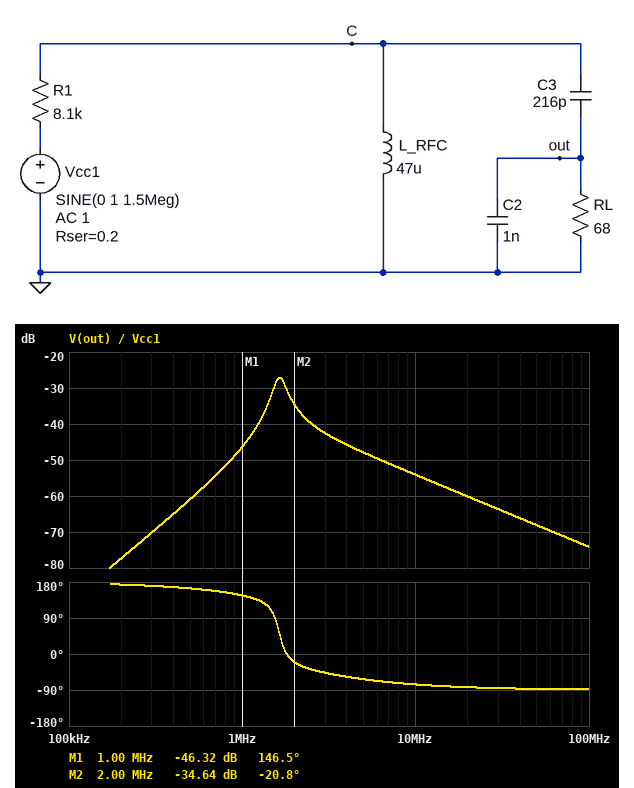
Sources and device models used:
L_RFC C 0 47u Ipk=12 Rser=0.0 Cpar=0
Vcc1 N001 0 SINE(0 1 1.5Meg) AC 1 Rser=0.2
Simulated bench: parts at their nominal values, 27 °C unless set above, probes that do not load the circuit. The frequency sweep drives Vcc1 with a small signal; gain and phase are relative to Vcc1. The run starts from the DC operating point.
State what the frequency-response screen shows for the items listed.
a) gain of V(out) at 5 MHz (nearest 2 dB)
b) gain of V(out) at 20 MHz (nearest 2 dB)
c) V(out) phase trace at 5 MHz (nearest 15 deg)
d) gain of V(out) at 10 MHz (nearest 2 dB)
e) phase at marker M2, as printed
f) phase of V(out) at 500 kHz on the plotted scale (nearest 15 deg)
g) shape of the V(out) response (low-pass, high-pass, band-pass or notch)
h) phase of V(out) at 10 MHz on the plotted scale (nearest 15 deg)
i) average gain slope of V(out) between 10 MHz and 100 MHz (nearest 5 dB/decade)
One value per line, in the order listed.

-48 dB
-60 dB
-60 deg
-54 dB
-20.8 deg
165 deg
band-pass
-75 deg
-20 dB/decade
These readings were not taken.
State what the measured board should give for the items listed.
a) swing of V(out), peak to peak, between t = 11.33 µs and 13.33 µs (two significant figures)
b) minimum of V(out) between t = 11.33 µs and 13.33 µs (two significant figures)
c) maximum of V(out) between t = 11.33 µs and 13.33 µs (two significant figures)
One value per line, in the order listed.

58 mV
-29 mV
29 mV
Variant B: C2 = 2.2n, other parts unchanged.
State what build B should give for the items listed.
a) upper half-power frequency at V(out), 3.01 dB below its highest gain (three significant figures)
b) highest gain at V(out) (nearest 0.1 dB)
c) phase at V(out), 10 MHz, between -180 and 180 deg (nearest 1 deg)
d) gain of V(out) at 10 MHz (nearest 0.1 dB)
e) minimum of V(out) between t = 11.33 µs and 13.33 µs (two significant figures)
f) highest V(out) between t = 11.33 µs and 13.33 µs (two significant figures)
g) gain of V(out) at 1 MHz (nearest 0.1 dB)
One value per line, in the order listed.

1.72 MHz
-26.9 dB
-83 deg
-60.8 dB
-23 mV
23 mV
-48.5 dB
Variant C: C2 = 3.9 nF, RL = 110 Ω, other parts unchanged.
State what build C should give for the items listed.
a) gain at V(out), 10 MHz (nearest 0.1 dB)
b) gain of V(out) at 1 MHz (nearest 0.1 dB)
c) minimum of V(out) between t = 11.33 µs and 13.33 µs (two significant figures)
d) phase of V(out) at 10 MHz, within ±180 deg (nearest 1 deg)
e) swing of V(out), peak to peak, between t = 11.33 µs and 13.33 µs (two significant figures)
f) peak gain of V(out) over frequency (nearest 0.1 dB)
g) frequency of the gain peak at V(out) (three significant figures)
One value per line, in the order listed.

-65.7 dB
-50.7 dB
-18 mV
-87 deg
36 mV
-27.3 dB
1.62 MHz
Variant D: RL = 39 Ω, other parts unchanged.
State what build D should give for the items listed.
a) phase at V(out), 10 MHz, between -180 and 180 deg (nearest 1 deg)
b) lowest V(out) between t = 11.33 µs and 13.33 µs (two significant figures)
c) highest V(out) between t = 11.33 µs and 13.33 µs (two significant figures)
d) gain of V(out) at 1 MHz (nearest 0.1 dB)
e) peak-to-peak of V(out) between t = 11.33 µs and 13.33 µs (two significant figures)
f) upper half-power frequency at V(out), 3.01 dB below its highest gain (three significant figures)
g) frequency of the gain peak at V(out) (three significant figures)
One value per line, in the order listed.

-67 deg
-23 mV
23 mV
-50.3 dB
47 mV
1.72 MHz
1.61 MHz
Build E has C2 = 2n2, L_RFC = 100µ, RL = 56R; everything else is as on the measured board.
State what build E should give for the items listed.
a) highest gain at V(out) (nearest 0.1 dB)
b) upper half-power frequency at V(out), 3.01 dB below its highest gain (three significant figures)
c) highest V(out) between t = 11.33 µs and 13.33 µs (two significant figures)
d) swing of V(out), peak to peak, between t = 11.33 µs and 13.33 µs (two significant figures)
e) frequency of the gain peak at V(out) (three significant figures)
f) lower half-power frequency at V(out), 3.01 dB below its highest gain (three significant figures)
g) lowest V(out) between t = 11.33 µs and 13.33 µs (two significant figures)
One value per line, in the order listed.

-28.0 dB
1.19 MHz
9.8 mV
20 mV
1.11 MHz
1.04 MHz
-9.8 mV
